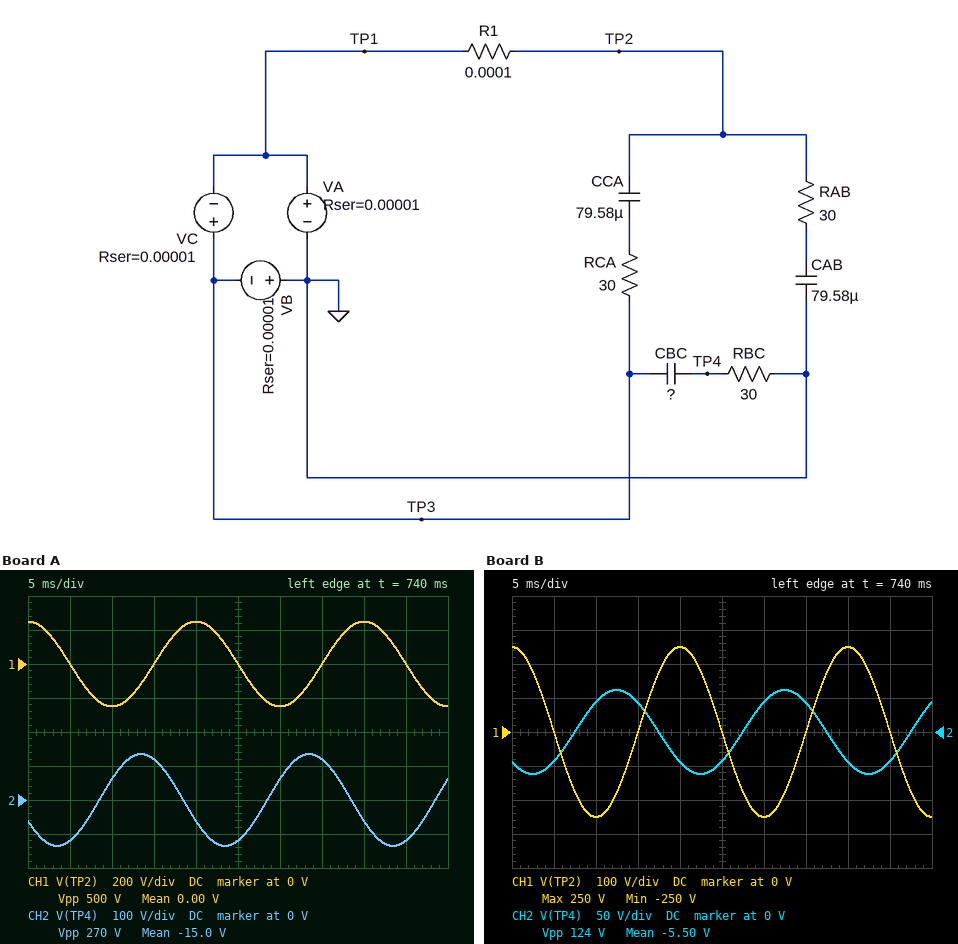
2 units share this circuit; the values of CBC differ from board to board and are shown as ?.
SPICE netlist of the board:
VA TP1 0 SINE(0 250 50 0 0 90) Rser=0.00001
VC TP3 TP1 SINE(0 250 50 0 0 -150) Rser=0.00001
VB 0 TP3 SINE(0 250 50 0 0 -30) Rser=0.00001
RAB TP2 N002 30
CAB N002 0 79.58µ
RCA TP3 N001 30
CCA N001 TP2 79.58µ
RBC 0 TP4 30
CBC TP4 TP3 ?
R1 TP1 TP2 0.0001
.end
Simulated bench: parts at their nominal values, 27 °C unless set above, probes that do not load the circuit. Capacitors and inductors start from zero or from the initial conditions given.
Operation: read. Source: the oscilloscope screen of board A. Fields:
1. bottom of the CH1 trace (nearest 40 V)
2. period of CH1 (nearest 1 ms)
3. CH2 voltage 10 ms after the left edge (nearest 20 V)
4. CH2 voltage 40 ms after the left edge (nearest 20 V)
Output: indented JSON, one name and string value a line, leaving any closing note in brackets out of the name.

{
  "bottom of the CH1 trace": "-240 V",
  "period of CH1": "20 ms",
  "CH2 voltage 10 ms after the left edge": "60 V",
  "CH2 voltage 40 ms after the left edge": "-60 V"
}
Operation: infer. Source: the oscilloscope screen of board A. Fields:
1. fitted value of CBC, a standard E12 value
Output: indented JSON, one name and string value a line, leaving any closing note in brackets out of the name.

{
  "fitted value of CBC, a standard E12 value": "68 µF"
}
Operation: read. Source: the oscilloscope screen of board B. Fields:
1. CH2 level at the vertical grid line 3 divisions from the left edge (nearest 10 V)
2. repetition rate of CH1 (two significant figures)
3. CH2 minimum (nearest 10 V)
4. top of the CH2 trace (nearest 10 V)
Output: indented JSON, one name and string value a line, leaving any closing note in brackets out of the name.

{
  "CH2 level at the vertical grid line 3 divisions from the left edge": "40 V",
  "repetition rate of CH1": "50 Hz",
  "CH2 minimum": "-60 V",
  "top of the CH2 trace": "60 V"
}
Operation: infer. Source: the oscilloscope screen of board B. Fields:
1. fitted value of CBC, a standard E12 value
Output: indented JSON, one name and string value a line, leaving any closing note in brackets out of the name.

{
  "fitted value of CBC, a standard E12 value": "27 µF"
}
